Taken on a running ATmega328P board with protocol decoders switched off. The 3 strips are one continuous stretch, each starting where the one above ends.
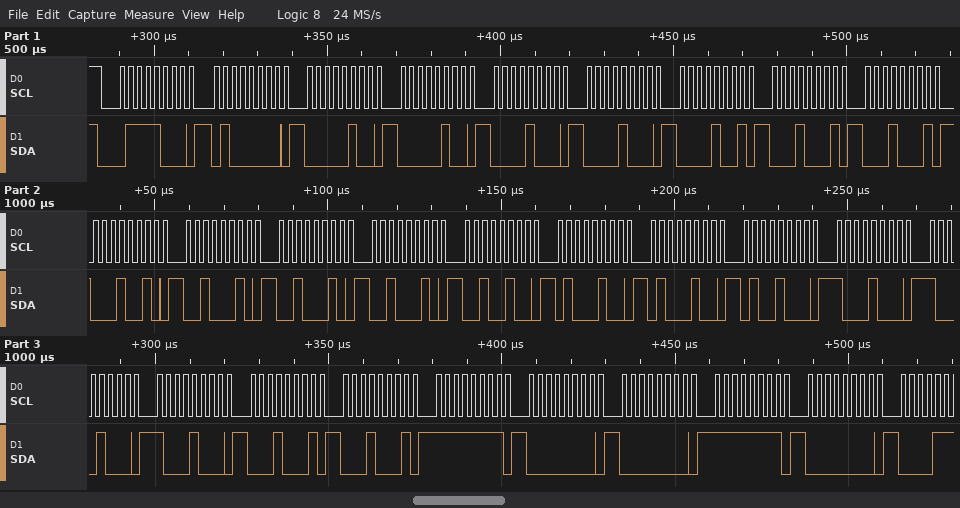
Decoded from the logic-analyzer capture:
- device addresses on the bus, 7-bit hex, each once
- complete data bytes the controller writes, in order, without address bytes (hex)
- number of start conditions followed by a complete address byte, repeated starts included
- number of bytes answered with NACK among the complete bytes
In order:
0x3C
40 04 04 08 08 09 11 11 12 22 22 22 24 44 44 48 88 88 88 11 11 FF 00 00 FF 00
1
0
